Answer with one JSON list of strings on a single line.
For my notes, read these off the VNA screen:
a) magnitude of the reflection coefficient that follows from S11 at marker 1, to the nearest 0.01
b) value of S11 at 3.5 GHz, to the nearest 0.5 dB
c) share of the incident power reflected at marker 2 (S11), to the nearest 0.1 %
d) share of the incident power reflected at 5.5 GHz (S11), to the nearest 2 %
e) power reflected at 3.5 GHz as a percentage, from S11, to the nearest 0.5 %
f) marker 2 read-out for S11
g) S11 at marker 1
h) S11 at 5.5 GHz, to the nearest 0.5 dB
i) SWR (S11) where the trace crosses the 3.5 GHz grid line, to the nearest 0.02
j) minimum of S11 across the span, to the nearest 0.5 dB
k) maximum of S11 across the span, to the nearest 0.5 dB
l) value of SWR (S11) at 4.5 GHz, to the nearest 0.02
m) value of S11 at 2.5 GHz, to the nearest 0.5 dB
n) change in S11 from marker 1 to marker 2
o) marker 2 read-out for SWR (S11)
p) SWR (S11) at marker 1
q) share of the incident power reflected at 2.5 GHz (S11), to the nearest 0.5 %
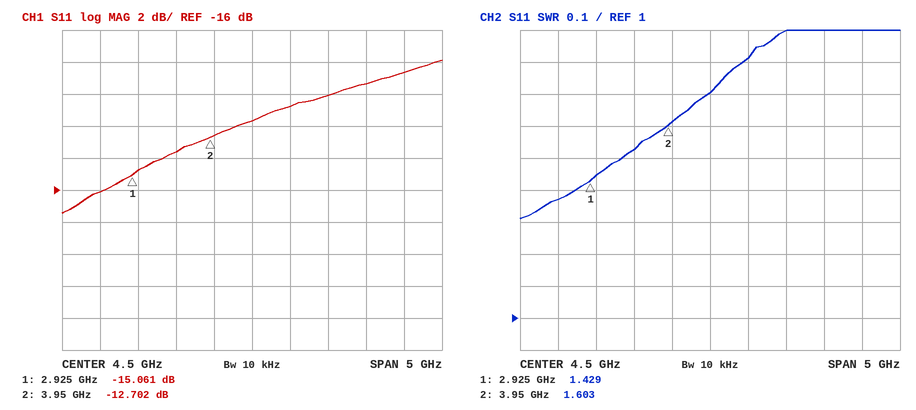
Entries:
["0.18", "-13.5 dB", "5.4 %", "10 %", "4.5 %", "-12.702 dB", "-15.061 dB", "-10.0 dB", "1.52", "-17.5 dB", "-8.0 dB", "1.70", "-16.0 dB", "2.359 dB", "1.603", "1.429", "2.5 %"]
